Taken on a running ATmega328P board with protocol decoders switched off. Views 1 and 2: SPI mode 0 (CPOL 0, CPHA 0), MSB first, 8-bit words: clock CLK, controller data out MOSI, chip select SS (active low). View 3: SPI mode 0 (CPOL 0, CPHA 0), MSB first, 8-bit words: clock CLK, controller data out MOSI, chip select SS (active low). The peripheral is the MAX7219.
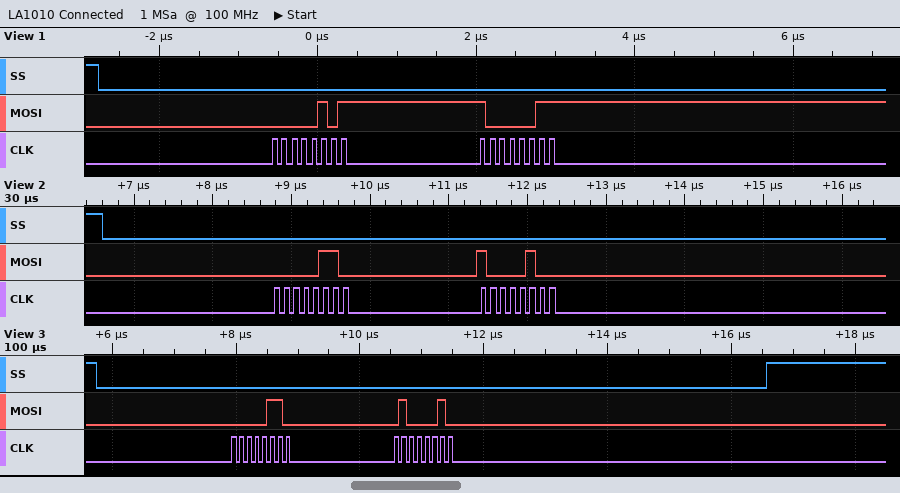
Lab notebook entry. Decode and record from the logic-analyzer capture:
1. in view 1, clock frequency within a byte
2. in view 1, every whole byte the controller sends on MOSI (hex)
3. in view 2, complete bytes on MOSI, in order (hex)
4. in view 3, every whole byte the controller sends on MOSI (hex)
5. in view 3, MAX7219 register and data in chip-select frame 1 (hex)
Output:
8 MHz
0x05 0x83
0x06 0x84
0x06 0x42
register 0x6, data 0x42
